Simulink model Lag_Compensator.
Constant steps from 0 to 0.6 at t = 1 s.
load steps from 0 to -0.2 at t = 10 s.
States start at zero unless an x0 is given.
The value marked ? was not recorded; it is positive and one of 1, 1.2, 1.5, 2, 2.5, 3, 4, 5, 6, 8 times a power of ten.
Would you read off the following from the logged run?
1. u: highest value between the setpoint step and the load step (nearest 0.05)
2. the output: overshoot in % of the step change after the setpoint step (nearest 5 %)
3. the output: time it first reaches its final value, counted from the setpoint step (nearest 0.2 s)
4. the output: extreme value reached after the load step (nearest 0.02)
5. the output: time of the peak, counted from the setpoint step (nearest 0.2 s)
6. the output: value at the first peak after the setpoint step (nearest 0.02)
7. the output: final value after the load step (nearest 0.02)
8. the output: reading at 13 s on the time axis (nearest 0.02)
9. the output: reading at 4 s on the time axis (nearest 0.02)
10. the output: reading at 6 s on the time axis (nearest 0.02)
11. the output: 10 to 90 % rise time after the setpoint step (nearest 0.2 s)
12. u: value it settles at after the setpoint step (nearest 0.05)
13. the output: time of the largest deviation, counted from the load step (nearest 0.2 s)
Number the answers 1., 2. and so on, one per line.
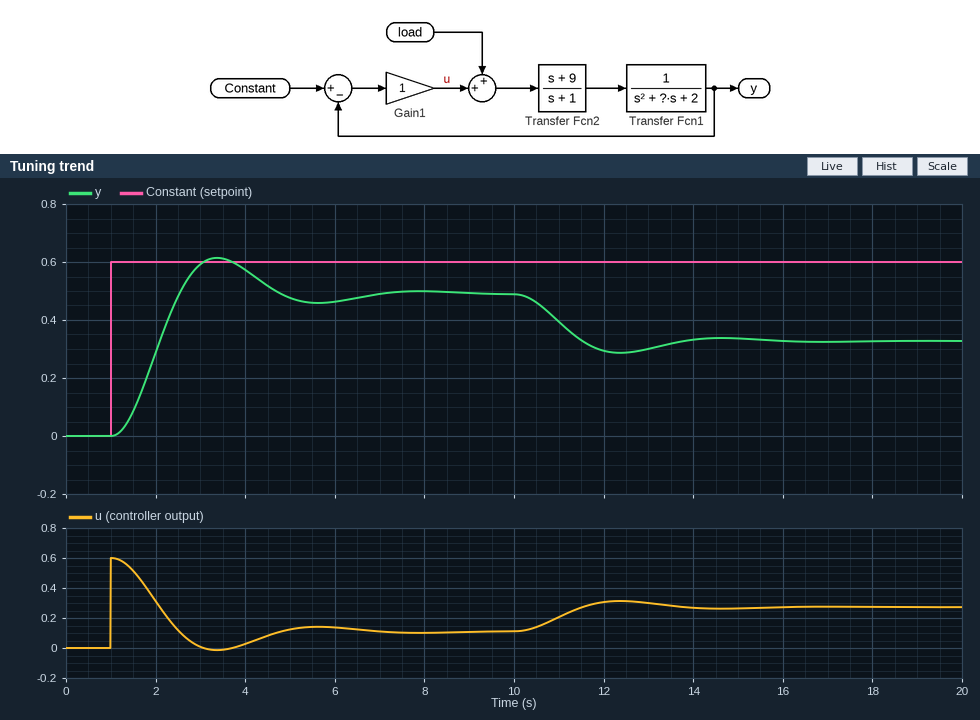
1. 0.60
2. 25 %
3. 1.6 s
4. 0.28
5. 2.4 s
6. 0.62
7. 0.32
8. 0.30
9. 0.58
10. 0.46
11. 1.0 s
12. 0.10
13. 2.4 s
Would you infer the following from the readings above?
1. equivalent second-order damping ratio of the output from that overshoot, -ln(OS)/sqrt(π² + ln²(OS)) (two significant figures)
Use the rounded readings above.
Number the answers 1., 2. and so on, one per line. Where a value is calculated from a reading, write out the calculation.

1. ln(0.25) = -1.386; 1.386 / sqrt(9.870 + 1.922) = 0.40
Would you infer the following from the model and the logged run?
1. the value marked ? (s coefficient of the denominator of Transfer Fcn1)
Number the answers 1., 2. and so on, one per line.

1. 5
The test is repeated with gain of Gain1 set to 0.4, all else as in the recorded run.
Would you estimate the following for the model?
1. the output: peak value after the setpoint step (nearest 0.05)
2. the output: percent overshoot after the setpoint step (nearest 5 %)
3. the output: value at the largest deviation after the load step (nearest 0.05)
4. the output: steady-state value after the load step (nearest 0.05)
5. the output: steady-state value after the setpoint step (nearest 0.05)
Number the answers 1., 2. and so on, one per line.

1. 0.40
2. 10 %
3. 0.05
4. 0.05
5. 0.40
